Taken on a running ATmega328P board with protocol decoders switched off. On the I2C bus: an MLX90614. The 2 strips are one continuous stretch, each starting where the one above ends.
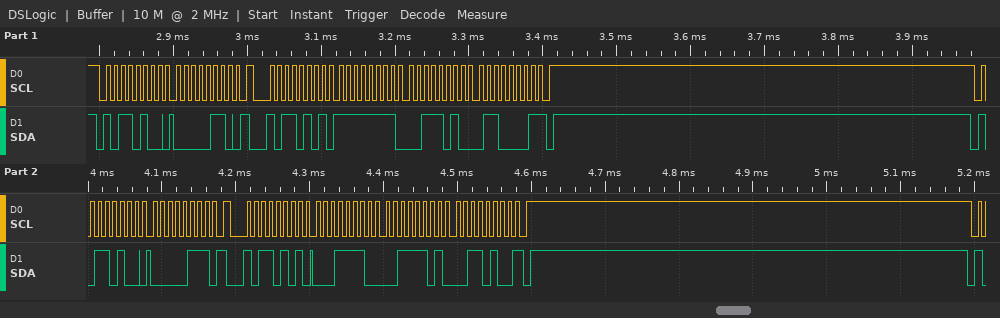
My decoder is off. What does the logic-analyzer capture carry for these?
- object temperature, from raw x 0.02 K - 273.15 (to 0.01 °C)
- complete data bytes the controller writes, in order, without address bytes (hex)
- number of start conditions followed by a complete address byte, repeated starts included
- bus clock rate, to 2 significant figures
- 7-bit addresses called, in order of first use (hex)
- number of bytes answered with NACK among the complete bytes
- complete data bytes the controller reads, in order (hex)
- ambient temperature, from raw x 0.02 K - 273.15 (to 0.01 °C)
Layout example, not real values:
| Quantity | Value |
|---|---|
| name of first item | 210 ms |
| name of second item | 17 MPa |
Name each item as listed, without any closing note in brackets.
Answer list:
| Quantity | Value |
|---|---|
| object temperature, from raw x 0.02 K - 273.15 | 39.77 °C |
| complete data bytes the controller writes, in order, without address bytes | 06 07 |
| number of start conditions followed by a complete address byte, repeated starts included | 4 |
| bus clock rate, to 2 significant figures | 100 kHz |
| 7-bit addresses called, in order of first use | 0x5A |
| number of bytes answered with NACK among the complete bytes | 2 |
| complete data bytes the controller reads, in order | FF 3A 61 1E 3D 34 |
| ambient temperature, from raw x 0.02 K - 273.15 | 28.91 °C |
